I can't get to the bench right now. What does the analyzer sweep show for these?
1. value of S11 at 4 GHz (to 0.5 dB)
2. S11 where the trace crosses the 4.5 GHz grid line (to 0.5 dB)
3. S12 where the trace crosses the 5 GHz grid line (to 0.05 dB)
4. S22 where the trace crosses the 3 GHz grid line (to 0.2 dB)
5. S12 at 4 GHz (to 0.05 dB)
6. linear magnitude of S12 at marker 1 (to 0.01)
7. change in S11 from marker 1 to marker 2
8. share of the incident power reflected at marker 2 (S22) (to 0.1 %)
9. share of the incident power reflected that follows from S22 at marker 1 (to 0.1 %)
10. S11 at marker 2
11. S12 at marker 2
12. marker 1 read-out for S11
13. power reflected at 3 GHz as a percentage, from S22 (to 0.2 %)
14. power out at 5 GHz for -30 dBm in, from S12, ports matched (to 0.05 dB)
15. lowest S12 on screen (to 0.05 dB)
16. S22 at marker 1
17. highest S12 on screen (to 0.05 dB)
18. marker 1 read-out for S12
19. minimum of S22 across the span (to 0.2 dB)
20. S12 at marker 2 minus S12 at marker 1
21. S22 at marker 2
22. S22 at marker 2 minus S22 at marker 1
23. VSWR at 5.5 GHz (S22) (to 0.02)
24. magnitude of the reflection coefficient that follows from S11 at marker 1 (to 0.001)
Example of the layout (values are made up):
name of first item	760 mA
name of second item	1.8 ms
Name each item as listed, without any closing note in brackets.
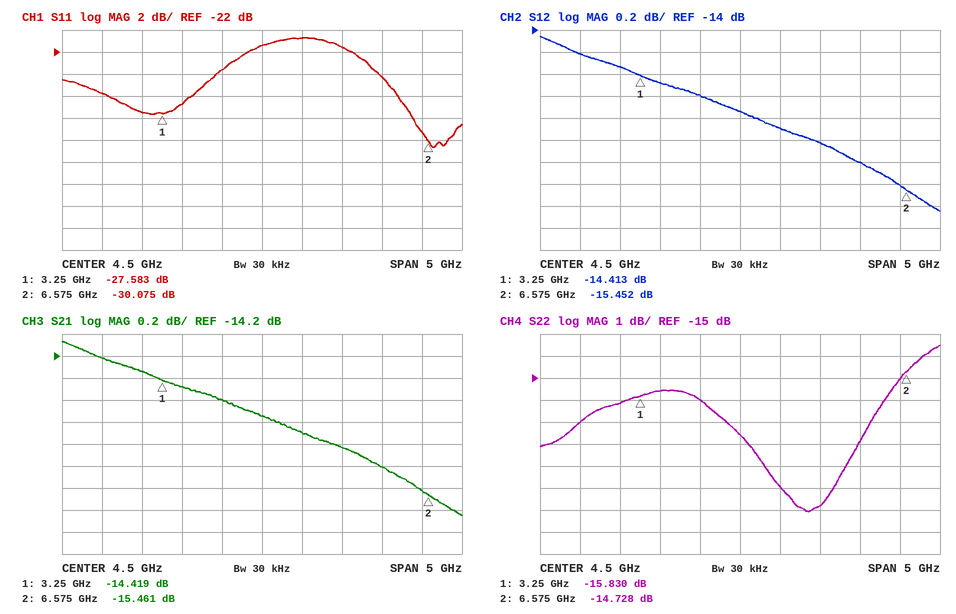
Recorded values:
value of S11 at 4 GHz	-23.5 dB
S11 where the trace crosses the 4.5 GHz grid line	-21.5 dB
S12 where the trace crosses the 5 GHz grid line	-14.90 dB
S22 where the trace crosses the 3 GHz grid line	-16.2 dB
S12 at 4 GHz	-14.60 dB
linear magnitude of S12 at marker 1	0.19
change in S11 from marker 1 to marker 2	-2.492 dB
share of the incident power reflected at marker 2 (S22)	3.4 %
share of the incident power reflected that follows from S22 at marker 1	2.6 %
S11 at marker 2	-30.075 dB
S12 at marker 2	-15.452 dB
marker 1 read-out for S11	-27.583 dB
power reflected at 3 GHz as a percentage, from S22	2.4 %
power out at 5 GHz for -30 dBm in, from S12, ports matched	-44.90 dBm
lowest S12 on screen	-15.65 dB
S22 at marker 1	-15.830 dB
highest S12 on screen	-14.05 dB
marker 1 read-out for S12	-14.413 dB
minimum of S22 across the span	-21.0 dB
S12 at marker 2 minus S12 at marker 1	-1.039 dB
S22 at marker 2	-14.728 dB
S22 at marker 2 minus S22 at marker 1	1.102 dB
VSWR at 5.5 GHz (S22)	1.20
magnitude of the reflection coefficient that follows from S11 at marker 1	0.042
